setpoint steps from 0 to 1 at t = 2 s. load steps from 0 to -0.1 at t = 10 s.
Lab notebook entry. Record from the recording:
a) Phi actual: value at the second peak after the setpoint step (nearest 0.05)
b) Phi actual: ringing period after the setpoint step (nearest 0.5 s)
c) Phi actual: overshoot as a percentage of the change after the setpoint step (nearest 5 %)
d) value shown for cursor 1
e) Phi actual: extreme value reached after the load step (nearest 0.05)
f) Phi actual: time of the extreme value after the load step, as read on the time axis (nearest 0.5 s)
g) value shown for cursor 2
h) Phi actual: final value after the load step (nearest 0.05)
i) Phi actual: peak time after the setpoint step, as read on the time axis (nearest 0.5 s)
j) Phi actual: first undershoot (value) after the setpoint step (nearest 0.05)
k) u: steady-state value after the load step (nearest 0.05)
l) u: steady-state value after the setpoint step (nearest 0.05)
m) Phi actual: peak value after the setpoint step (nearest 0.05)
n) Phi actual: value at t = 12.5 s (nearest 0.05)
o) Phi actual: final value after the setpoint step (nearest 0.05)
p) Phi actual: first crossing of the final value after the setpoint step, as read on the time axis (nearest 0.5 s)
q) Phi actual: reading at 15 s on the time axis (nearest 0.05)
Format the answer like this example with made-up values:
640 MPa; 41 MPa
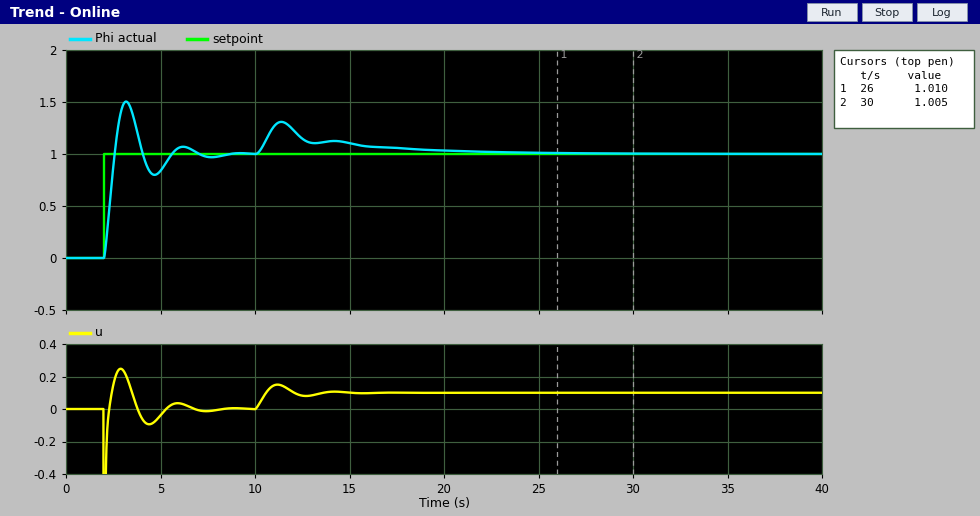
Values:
1.05; 3.0 s; 50 %; 1.010; 1.30; 11.5 s; 1.005; 1.00; 3.0 s; 0.80; 0.10; 0.00; 1.50; 1.15; 1.00; 2.5 s; 1.10
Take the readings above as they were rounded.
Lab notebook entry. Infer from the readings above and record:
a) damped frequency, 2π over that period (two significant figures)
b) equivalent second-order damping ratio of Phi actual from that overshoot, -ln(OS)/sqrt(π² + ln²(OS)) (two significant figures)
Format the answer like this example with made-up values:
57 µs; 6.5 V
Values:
2.1 rad/s; 0.22
